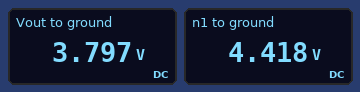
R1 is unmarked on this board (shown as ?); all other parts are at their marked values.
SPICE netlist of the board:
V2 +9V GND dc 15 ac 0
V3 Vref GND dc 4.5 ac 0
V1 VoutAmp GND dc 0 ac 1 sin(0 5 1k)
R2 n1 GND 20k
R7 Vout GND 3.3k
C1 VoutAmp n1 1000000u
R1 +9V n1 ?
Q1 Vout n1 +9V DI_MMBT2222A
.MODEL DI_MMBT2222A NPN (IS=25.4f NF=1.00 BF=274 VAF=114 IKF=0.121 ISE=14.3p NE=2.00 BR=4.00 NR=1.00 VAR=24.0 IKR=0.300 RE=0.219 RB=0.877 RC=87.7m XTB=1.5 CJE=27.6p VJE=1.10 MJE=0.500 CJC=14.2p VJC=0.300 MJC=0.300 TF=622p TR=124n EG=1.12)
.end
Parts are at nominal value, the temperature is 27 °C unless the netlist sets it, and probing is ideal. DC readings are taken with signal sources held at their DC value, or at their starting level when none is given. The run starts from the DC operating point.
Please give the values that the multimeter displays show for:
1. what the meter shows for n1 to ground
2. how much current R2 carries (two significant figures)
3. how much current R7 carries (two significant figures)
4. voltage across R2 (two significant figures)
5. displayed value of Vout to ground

4.418 V
220 µA
1.2 mA
4.4 V
3.797 V
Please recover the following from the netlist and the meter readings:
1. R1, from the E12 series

27 kΩ
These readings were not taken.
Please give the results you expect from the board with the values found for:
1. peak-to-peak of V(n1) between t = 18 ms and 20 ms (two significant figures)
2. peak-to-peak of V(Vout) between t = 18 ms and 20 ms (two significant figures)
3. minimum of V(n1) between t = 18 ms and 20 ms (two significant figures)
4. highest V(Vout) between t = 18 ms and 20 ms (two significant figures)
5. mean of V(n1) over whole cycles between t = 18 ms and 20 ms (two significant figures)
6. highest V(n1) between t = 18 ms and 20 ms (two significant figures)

10 V
8.8 V
-580 mV
8.8 V
4.4 V
9.4 V
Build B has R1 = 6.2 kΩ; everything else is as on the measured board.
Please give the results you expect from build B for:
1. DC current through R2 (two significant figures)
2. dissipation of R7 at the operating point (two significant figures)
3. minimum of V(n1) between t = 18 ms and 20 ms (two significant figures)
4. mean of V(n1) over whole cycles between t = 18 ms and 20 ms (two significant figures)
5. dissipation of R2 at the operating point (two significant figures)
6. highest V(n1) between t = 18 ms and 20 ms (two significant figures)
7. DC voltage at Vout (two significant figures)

470 µA
23 mW
4.3 V
9.3 V
4.4 mW
14 V
8.7 V
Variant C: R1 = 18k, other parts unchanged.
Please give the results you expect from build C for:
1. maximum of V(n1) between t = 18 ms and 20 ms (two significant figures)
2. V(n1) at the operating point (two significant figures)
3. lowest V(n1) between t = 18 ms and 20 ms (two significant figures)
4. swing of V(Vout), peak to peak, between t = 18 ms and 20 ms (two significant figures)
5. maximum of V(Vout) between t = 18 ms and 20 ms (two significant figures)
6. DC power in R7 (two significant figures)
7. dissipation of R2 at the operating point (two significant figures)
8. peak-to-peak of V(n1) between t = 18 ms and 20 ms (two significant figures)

11 V
5.7 V
670 mV
9.9 V
10 V
7.7 mW
1.6 mW
10 V
